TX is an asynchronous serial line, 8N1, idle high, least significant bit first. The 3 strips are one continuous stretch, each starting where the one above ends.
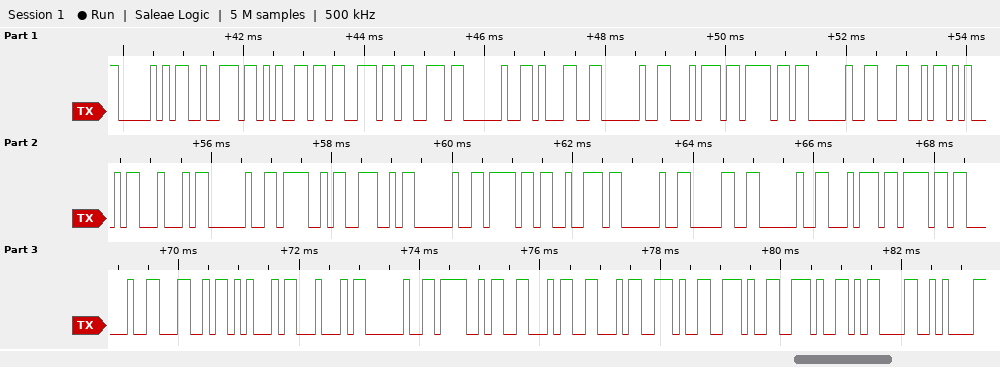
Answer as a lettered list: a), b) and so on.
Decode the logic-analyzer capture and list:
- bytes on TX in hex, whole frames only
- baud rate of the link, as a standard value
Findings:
a) 50 72 65 73 73 20 31 20 74 6F 20 4C 45 44 20 4F 4E 20 6F 72 20 30 20 74 6F 20 4C 45 44 20 4F 46 46 2E 2E 2E 0D 0A
b) 9600 baud
